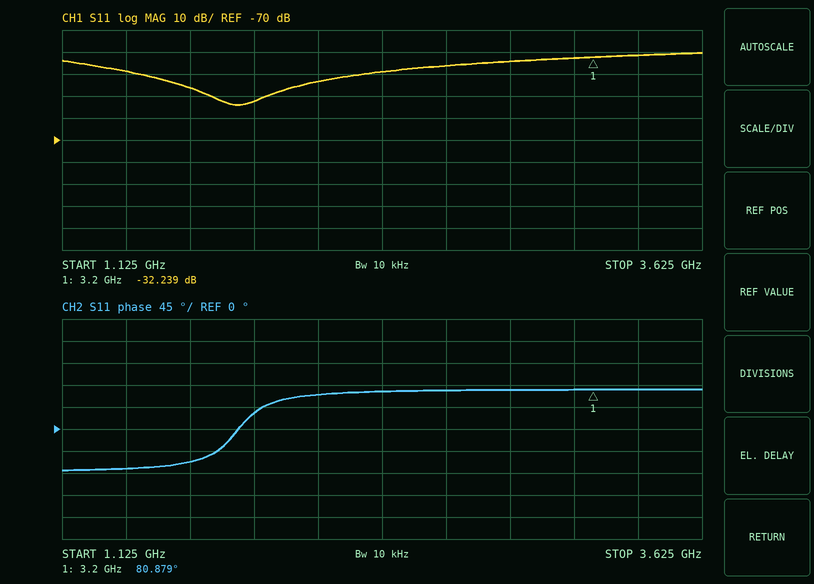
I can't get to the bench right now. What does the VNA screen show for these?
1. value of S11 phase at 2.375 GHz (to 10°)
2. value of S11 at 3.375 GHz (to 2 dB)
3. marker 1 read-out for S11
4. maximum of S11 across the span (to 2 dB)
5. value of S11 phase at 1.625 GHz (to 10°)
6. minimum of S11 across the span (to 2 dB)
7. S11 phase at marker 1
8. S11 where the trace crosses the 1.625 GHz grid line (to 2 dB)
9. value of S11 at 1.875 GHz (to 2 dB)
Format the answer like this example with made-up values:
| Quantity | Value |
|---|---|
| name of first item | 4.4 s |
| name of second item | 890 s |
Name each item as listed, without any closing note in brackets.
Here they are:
| Quantity | Value |
|---|---|
| value of S11 phase at 2.375 GHz | 80° |
| value of S11 at 3.375 GHz | -32 dB |
| marker 1 read-out for S11 | -32.239 dB |
| maximum of S11 across the span | -30 dB |
| value of S11 phase at 1.625 GHz | -70° |
| minimum of S11 across the span | -54 dB |
| S11 phase at marker 1 | 80.879° |
| S11 where the trace crosses the 1.625 GHz grid line | -46 dB |
| value of S11 at 1.875 GHz | -52 dB |
